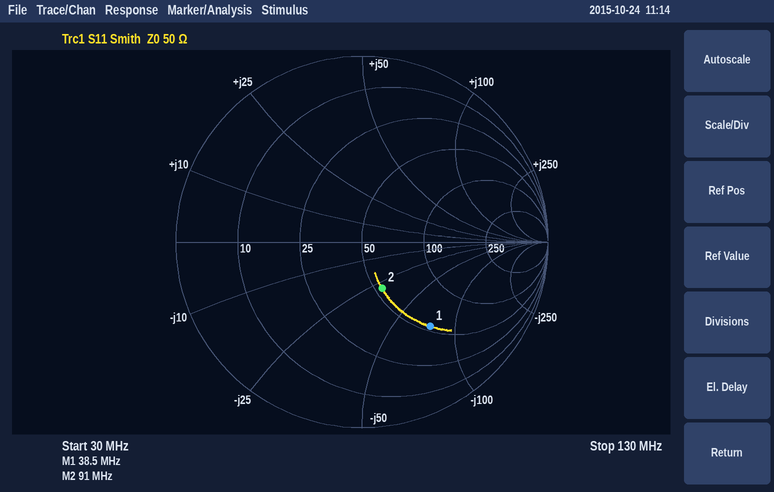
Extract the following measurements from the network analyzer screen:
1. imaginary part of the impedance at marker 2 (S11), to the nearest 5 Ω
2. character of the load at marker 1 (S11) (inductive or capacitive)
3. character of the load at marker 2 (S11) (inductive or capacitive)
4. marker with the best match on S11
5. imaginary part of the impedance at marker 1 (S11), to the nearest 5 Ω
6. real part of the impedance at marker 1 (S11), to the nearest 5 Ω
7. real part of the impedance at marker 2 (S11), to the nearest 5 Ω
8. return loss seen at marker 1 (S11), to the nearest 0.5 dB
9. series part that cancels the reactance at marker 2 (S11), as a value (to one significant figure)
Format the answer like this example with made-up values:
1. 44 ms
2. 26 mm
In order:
1. -30 Ω
2. capacitive
3. capacitive
4. marker 2
5. -75 Ω
6. 55 Ω
7. 55 Ω
8. 4.5 dB
9. 50 nH
